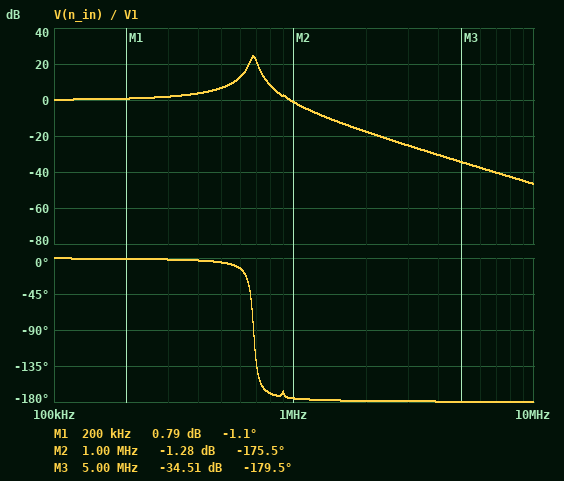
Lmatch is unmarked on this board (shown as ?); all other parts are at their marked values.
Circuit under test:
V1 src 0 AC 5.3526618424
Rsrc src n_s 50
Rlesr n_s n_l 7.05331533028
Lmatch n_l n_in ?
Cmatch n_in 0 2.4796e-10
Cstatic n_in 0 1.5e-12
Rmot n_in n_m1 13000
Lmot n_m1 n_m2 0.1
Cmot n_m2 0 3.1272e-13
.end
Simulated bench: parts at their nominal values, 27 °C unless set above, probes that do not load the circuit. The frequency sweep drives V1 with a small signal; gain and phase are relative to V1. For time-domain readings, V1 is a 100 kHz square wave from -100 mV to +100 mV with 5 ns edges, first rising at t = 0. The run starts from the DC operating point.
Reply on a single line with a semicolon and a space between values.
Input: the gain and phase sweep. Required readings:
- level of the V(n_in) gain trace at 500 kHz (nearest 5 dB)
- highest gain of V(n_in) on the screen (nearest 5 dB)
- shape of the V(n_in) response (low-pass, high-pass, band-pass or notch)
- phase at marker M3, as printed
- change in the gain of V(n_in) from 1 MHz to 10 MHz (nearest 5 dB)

5 dB; 25 dB; low-pass; -179.5 deg; -45 dB
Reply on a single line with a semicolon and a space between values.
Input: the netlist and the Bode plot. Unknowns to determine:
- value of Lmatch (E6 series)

220 µH
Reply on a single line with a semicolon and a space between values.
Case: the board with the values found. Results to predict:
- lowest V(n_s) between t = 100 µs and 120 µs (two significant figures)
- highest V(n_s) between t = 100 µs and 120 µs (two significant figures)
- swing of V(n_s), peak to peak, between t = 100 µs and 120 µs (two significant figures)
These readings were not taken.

-110 mV; 110 mV; 230 mV
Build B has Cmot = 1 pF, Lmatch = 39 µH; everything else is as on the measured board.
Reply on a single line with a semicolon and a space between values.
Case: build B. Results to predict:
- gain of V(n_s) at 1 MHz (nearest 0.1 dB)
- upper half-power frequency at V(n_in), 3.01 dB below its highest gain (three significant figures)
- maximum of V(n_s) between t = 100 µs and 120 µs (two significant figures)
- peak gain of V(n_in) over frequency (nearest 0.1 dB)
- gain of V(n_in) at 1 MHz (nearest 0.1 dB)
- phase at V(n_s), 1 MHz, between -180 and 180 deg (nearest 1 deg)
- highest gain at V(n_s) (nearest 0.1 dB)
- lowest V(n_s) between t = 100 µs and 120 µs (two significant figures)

-0.1 dB; 1.72 MHz; 120 mV; 16.8 dB; 4.1 dB; -7 deg; 0 dB; -120 mV
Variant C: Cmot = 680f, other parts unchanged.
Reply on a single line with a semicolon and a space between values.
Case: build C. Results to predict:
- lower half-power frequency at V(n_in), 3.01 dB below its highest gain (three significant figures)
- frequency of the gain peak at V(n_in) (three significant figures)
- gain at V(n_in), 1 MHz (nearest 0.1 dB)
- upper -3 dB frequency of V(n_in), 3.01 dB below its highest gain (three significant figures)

663 kHz; 683 kHz; -1.3 dB; 703 kHz
